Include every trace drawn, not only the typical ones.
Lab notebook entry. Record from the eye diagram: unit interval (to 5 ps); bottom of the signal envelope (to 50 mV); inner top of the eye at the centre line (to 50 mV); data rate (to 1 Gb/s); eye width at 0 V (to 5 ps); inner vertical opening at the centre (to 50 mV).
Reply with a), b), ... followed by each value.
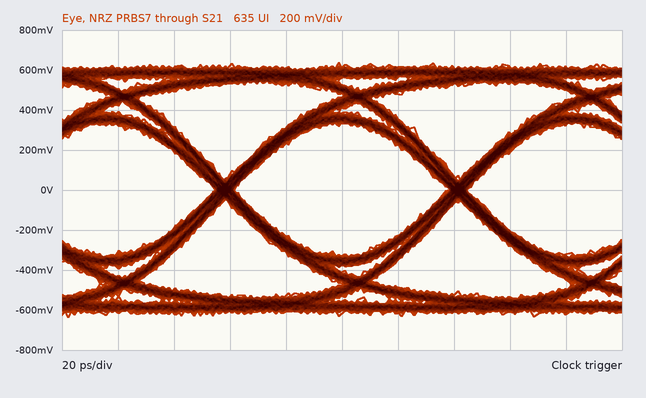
a) 85 ps
b) -650 mV
c) 350 mV
d) 12 Gb/s
e) 75 ps
f) 650 mV
